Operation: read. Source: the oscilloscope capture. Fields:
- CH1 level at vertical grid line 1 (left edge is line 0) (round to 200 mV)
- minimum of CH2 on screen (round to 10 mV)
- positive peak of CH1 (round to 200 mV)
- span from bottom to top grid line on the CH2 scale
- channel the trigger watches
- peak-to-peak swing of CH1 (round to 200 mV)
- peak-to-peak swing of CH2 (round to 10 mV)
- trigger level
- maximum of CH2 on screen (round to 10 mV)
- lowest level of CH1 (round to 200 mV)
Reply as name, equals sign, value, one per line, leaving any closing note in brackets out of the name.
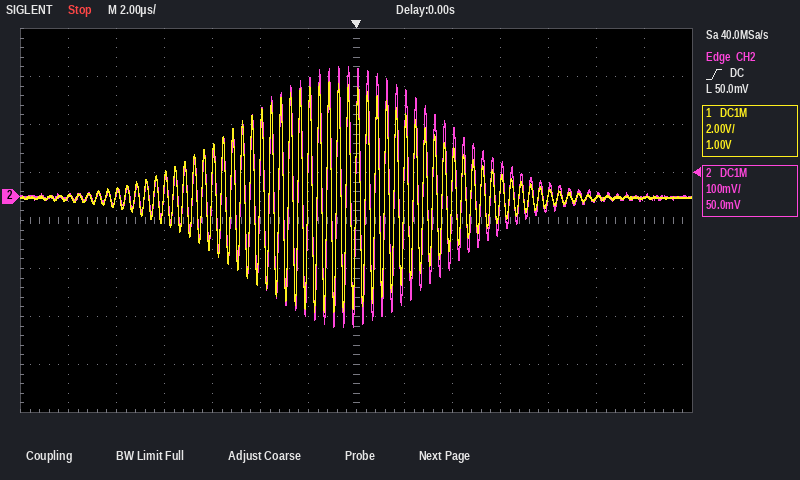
CH1 level at vertical grid line 1 (left edge is line 0) = 0.0 V
minimum of CH2 on screen = -270 mV
positive peak of CH1 = 4.8 V
span from bottom to top grid line on the CH2 scale = 800 mV
channel the trigger watches = CH2
peak-to-peak swing of CH1 = 9.6 V
peak-to-peak swing of CH2 = 540 mV
trigger level = 50.0 mV
maximum of CH2 on screen = 270 mV
lowest level of CH1 = -4.8 V
